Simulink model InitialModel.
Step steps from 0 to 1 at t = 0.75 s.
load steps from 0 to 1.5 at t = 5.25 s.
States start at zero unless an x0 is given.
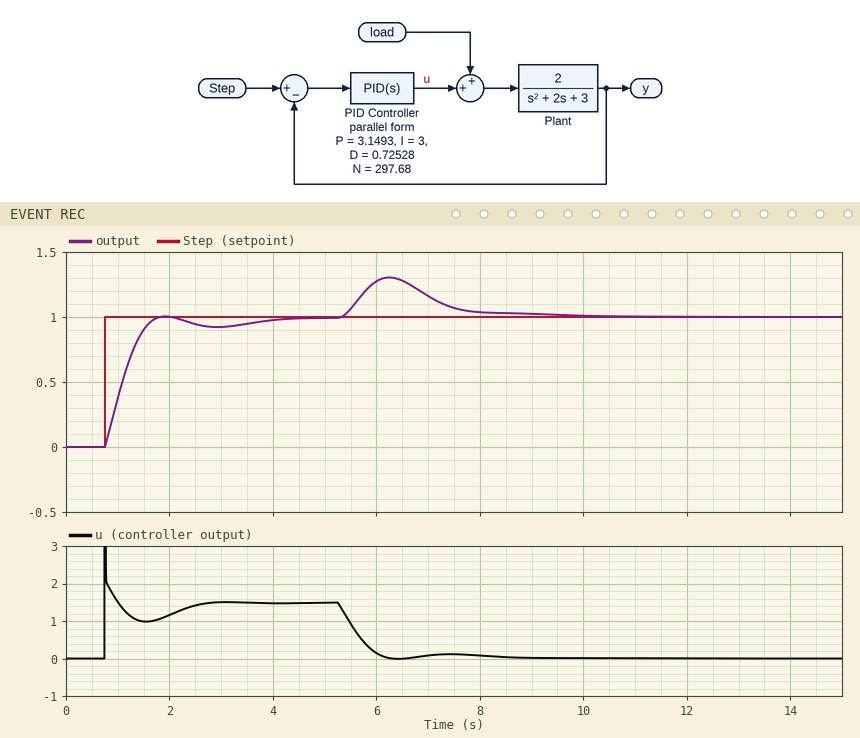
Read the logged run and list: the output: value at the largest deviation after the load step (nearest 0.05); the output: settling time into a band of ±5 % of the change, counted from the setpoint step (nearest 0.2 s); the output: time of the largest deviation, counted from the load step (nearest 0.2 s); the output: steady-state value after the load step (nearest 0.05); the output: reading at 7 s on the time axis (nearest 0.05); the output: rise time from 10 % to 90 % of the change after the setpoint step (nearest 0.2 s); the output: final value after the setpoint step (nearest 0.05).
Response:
1.30
2.8 s
1.0 s
1.00
1.15
0.6 s
1.00
